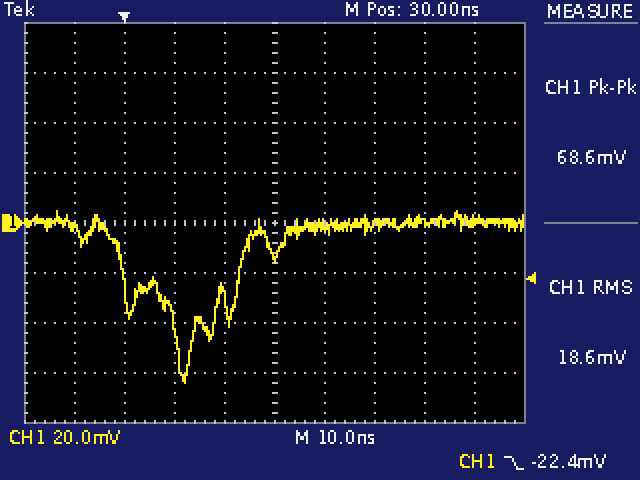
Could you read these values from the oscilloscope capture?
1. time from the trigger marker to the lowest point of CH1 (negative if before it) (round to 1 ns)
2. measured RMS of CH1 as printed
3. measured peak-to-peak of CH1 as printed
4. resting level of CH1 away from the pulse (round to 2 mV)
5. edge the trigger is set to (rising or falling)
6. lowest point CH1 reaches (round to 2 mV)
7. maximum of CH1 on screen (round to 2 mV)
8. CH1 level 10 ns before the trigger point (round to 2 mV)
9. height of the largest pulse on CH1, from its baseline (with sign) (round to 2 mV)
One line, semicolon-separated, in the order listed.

+12 ns; 18.6 mV; 68.6 mV; 0 mV; falling; -64 mV; 4 mV; -2 mV; -64 mV
